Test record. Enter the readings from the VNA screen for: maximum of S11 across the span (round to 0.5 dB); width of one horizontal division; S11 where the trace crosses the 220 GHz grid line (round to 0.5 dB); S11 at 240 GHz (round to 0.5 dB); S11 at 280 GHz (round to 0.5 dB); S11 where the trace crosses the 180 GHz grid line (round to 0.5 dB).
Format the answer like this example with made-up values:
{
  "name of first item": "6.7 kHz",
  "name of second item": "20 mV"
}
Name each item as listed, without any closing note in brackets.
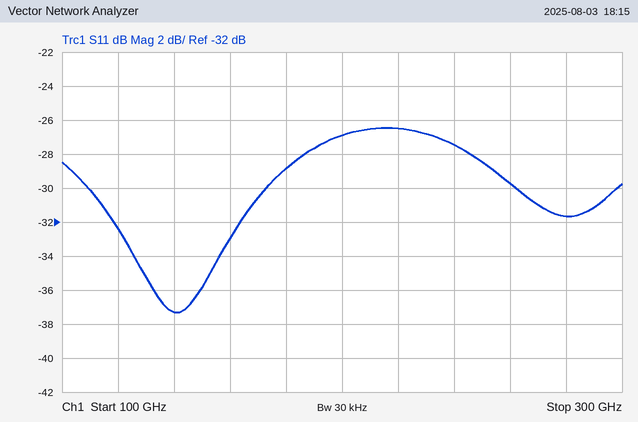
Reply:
{
  "maximum of S11 across the span": "-26.5 dB",
  "width of one horizontal division": "20 GHz",
  "S11 where the trace crosses the 220 GHz grid line": "-26.5 dB",
  "S11 at 240 GHz": "-27.5 dB",
  "S11 at 280 GHz": "-31.5 dB",
  "S11 where the trace crosses the 180 GHz grid line": "-29.0 dB"
}
